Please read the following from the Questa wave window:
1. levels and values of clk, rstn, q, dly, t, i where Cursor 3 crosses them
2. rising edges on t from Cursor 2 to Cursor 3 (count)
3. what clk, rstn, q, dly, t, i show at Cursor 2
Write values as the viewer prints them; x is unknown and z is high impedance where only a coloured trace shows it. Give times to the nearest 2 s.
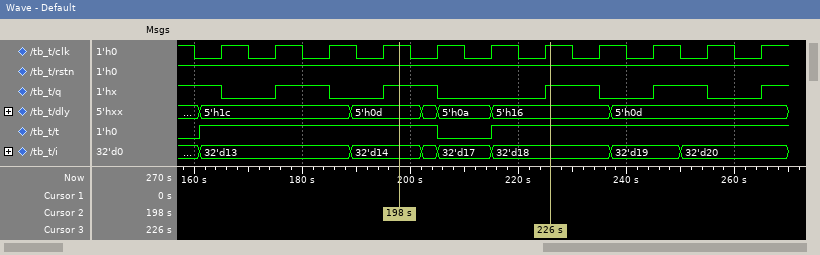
clk=1, rstn=1, q=1, dly=5'h16, t=1, i=32'd18
1
clk=1, rstn=1, q=1, dly=5'h0d, t=1, i=32'd14
